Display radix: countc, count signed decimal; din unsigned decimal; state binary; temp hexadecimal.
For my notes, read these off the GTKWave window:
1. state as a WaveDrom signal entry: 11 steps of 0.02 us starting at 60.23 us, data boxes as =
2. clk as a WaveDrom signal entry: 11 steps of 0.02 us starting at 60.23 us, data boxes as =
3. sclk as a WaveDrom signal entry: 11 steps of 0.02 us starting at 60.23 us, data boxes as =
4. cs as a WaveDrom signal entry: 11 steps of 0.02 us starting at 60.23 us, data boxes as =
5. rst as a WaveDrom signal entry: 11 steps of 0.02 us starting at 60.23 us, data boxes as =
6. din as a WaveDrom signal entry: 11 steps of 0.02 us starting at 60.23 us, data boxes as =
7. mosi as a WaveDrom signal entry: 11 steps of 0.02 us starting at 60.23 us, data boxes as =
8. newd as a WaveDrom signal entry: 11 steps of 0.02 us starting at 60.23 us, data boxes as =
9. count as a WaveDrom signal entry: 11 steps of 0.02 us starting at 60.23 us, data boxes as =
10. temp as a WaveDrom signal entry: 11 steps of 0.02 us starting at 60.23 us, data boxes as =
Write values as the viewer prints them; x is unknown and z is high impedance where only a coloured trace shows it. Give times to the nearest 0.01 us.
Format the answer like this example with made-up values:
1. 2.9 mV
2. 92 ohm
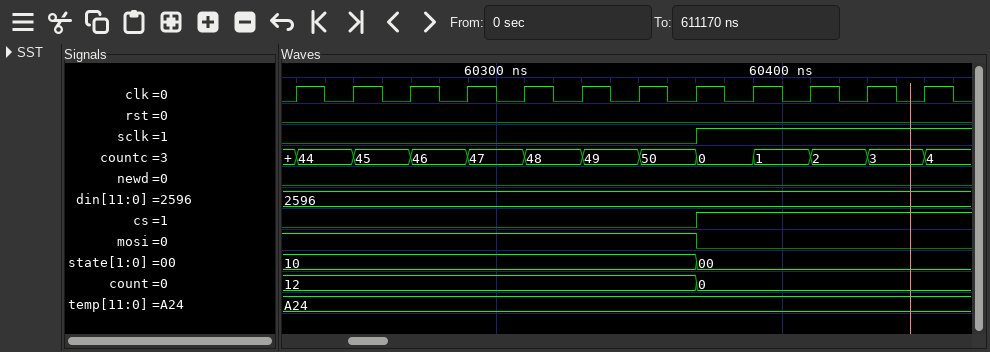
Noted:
1. {name: 'state', wave: '=......=...', data: '10 00'}
2. {name: 'clk', wave: 'p..........'}
3. {name: 'sclk', wave: '0......1...'}
4. {name: 'cs', wave: '0......1...'}
5. {name: 'rst', wave: '0..........'}
6. {name: 'din', wave: '=..........', data: '2596'}
7. {name: 'mosi', wave: '1......0...'}
8. {name: 'newd', wave: '0..........'}
9. {name: 'count', wave: '=......=...', data: '12 0'}
10. {name: 'temp', wave: '=..........', data: 'A24'}
